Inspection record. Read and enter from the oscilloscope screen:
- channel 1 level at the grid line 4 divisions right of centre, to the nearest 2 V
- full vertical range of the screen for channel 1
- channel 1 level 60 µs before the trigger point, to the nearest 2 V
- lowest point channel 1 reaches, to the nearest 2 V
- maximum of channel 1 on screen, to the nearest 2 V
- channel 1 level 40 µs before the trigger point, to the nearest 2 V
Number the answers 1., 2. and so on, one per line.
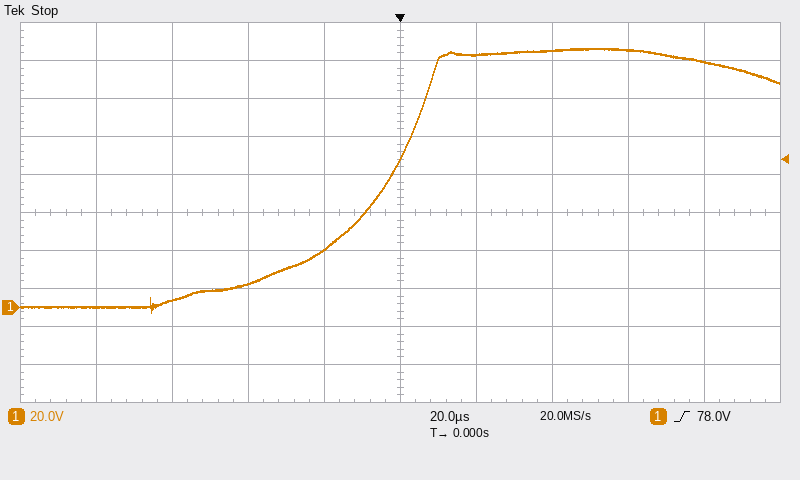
1. 130 V
2. 200 V
3. 4 V
4. -2 V
5. 136 V
6. 12 V
